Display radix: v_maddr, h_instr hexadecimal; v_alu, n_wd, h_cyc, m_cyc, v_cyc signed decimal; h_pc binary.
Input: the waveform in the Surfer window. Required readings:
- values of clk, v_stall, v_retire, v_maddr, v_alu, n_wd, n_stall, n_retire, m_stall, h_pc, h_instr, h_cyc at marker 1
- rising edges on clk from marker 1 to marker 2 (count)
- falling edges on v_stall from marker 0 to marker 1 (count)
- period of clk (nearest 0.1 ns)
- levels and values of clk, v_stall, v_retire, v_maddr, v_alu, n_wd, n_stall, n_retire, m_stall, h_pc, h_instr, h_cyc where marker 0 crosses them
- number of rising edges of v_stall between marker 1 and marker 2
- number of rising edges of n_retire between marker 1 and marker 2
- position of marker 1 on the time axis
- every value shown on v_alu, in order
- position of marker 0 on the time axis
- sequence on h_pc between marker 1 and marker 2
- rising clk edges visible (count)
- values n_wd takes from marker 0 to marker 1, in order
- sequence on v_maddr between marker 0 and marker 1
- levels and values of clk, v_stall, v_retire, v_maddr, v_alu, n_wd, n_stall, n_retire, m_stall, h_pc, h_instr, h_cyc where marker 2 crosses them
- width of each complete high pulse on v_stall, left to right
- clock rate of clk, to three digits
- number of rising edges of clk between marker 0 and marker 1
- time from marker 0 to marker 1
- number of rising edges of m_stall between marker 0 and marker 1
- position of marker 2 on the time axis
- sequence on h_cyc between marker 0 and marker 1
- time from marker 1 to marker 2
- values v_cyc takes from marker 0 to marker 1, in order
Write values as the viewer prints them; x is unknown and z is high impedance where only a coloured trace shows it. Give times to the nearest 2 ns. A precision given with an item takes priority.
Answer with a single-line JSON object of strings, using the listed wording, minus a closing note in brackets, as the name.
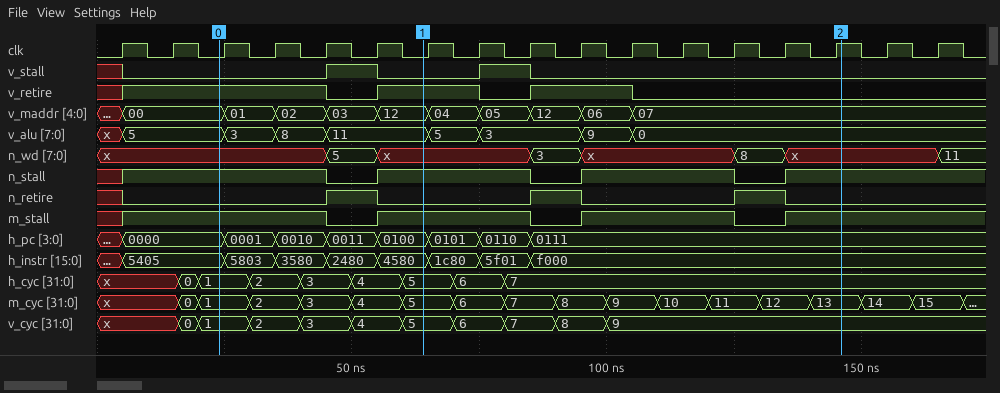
{"values of clk, v_stall, v_retire, v_maddr, v_alu, n_wd, n_stall, n_retire, m_stall, h_pc, h_instr, h_cyc at marker 1": "clk=0, v_stall=0, v_retire=1, v_maddr=12, v_alu=11, n_wd=x, n_stall=1, n_retire=0, m_stall=1, h_pc=0100, h_instr=4580, h_cyc=5", "rising edges on clk from marker 1 to marker 2": "9", "falling edges on v_stall from marker 0 to marker 1": "1", "period of clk": "10 ns", "levels and values of clk, v_stall, v_retire, v_maddr, v_alu, n_wd, n_stall, n_retire, m_stall, h_pc, h_instr, h_cyc where marker 0 crosses them": "clk=0, v_stall=0, v_retire=1, v_maddr=00, v_alu=5, n_wd=x, n_stall=1, n_retire=0, m_stall=1, h_pc=0000, h_instr=5405, h_cyc=1", "number of rising edges of v_stall between marker 1 and marker 2": "1", "number of rising edges of n_retire between marker 1 and marker 2": "2", "position of marker 1 on the time axis": "64 ns", "every value shown on v_alu, in order": "x, 5, 3, 8, 11, 5, 3, 9, 0", "position of marker 0 on the time axis": "24 ns", "sequence on h_pc between marker 1 and marker 2": "0100, 0101, 0110, 0111", "rising clk edges visible": "17", "values n_wd takes from marker 0 to marker 1, in order": "x, 5, x", "sequence on v_maddr between marker 0 and marker 1": "00, 01, 02, 03, 12", "levels and values of clk, v_stall, v_retire, v_maddr, v_alu, n_wd, n_stall, n_retire, m_stall, h_pc, h_instr, h_cyc where marker 2 crosses them": "clk=1, v_stall=0, v_retire=0, v_maddr=07, v_alu=0, n_wd=x, n_stall=1, n_retire=0, m_stall=1, h_pc=0111, h_instr=f000, h_cyc=7", "width of each complete high pulse on v_stall, left to right": "10 ns, 10 ns", "clock rate of clk, to three digits": "100 MHz", "number of rising edges of clk between marker 0 and marker 1": "4", "time from marker 0 to marker 1": "40 ns", "number of rising edges of m_stall between marker 0 and marker 1": "1", "position of marker 2 on the time axis": "146 ns", "sequence on h_cyc between marker 0 and marker 1": "1, 2, 3, 4, 5", "time from marker 1 to marker 2": "82 ns", "values v_cyc takes from marker 0 to marker 1, in order": "1, 2, 3, 4, 5"}
